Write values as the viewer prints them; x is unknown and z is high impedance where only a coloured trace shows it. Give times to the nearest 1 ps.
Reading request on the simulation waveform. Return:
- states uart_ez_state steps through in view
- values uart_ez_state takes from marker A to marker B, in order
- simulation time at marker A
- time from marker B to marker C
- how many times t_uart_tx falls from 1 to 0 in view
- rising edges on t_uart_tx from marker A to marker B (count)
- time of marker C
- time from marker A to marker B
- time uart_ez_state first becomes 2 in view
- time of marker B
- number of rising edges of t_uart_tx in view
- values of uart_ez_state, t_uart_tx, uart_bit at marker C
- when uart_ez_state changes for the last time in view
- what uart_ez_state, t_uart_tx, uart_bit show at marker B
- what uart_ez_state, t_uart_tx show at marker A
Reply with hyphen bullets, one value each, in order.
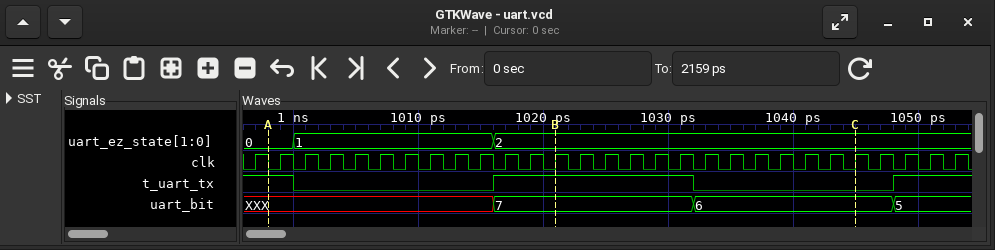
- 0, 1, 2
- 0, 1, 2
- 998 ps
- 24 ps
- 2
- 1
- 1045 ps
- 23 ps
- 1016 ps
- 1021 ps
- 2
- uart_ez_state=2, t_uart_tx=0, uart_bit=6
- 1016 ps
- uart_ez_state=2, t_uart_tx=1, uart_bit=7
- uart_ez_state=0, t_uart_tx=1
